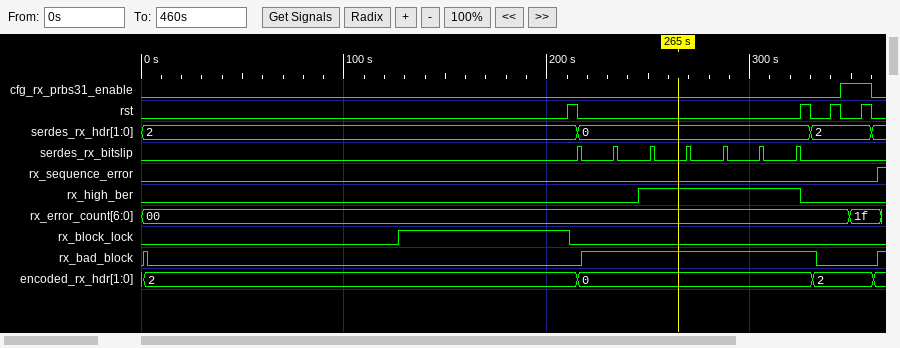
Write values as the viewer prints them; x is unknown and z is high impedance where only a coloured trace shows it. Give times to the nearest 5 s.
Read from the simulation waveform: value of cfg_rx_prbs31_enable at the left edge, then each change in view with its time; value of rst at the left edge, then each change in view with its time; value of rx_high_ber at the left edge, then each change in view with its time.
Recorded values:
0, 1 at 345 s, 0 at 360 s
0, 1 at 210 s, 0 at 215 s, 1 at 325 s, 0 at 330 s, 1 at 340 s, 0 at 345 s, 1 at 355 s, 0 at 360 s
0, 1 at 245 s, 0 at 325 s
